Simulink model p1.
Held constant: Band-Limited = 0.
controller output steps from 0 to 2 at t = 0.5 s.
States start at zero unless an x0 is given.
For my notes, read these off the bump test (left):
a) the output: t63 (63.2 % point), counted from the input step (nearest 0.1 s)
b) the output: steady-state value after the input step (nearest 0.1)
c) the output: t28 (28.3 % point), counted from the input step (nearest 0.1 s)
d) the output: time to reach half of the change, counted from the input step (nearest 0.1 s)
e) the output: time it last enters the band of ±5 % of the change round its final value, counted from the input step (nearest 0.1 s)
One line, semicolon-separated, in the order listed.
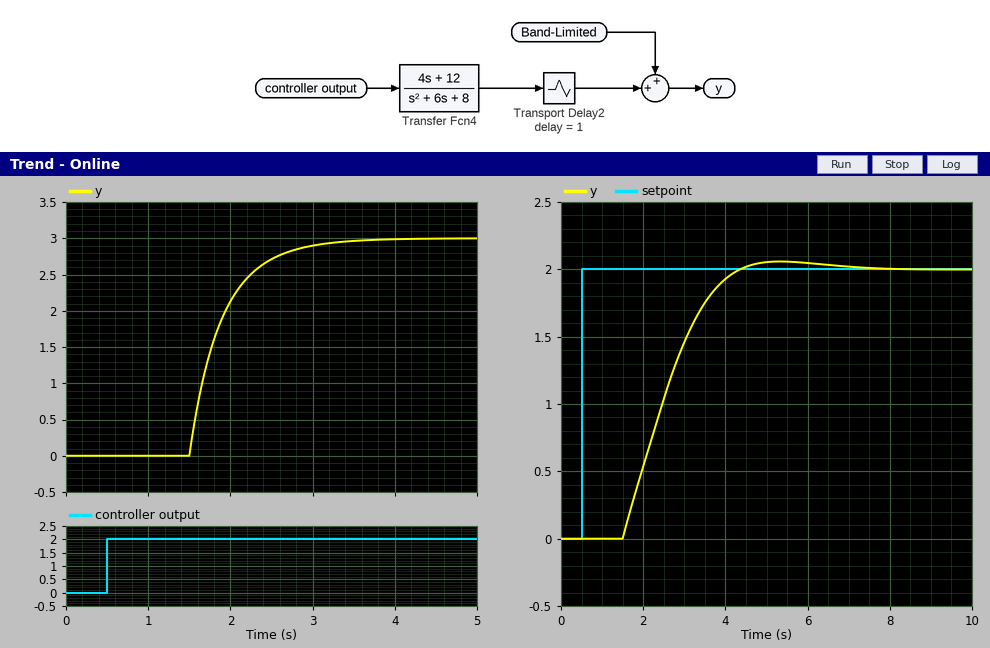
1.4 s; 3.0; 1.1 s; 1.3 s; 2.3 s
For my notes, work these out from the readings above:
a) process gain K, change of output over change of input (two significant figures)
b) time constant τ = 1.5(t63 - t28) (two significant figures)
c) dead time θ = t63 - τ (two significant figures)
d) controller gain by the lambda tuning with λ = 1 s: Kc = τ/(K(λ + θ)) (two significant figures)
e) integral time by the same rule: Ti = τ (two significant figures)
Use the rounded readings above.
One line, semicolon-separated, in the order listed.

1.5; 0.45 s; 0.95 s; 0.15; 0.45 s
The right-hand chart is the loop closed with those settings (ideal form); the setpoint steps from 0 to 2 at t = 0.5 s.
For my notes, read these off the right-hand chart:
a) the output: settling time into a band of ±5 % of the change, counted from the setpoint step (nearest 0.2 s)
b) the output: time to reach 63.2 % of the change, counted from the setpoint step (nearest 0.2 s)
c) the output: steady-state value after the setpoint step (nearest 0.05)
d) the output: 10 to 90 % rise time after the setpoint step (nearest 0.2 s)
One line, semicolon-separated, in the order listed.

3.4 s; 2.2 s; 2.00; 2.0 s
